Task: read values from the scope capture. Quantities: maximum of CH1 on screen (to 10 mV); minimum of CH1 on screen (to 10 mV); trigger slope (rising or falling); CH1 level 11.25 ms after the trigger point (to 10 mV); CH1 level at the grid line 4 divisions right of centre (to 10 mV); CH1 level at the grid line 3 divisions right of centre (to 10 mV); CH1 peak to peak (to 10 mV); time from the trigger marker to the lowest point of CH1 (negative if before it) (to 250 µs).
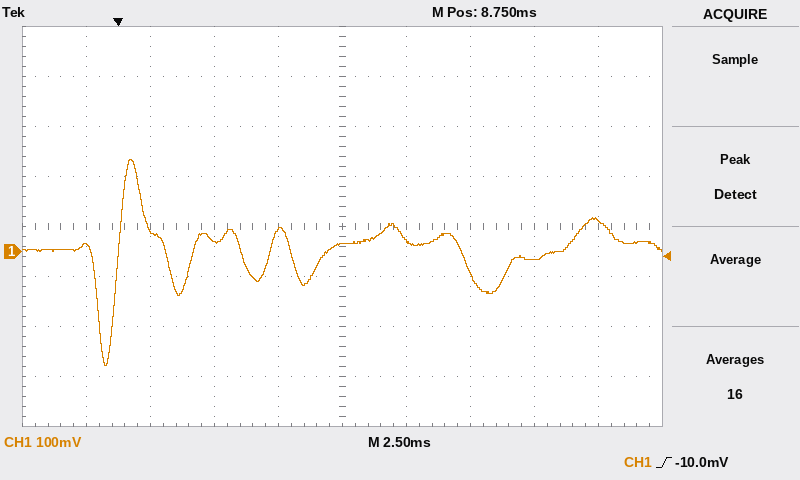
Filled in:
180 mV
-230 mV
rising
20 mV
60 mV
-20 mV
410 mV
-500 µs
